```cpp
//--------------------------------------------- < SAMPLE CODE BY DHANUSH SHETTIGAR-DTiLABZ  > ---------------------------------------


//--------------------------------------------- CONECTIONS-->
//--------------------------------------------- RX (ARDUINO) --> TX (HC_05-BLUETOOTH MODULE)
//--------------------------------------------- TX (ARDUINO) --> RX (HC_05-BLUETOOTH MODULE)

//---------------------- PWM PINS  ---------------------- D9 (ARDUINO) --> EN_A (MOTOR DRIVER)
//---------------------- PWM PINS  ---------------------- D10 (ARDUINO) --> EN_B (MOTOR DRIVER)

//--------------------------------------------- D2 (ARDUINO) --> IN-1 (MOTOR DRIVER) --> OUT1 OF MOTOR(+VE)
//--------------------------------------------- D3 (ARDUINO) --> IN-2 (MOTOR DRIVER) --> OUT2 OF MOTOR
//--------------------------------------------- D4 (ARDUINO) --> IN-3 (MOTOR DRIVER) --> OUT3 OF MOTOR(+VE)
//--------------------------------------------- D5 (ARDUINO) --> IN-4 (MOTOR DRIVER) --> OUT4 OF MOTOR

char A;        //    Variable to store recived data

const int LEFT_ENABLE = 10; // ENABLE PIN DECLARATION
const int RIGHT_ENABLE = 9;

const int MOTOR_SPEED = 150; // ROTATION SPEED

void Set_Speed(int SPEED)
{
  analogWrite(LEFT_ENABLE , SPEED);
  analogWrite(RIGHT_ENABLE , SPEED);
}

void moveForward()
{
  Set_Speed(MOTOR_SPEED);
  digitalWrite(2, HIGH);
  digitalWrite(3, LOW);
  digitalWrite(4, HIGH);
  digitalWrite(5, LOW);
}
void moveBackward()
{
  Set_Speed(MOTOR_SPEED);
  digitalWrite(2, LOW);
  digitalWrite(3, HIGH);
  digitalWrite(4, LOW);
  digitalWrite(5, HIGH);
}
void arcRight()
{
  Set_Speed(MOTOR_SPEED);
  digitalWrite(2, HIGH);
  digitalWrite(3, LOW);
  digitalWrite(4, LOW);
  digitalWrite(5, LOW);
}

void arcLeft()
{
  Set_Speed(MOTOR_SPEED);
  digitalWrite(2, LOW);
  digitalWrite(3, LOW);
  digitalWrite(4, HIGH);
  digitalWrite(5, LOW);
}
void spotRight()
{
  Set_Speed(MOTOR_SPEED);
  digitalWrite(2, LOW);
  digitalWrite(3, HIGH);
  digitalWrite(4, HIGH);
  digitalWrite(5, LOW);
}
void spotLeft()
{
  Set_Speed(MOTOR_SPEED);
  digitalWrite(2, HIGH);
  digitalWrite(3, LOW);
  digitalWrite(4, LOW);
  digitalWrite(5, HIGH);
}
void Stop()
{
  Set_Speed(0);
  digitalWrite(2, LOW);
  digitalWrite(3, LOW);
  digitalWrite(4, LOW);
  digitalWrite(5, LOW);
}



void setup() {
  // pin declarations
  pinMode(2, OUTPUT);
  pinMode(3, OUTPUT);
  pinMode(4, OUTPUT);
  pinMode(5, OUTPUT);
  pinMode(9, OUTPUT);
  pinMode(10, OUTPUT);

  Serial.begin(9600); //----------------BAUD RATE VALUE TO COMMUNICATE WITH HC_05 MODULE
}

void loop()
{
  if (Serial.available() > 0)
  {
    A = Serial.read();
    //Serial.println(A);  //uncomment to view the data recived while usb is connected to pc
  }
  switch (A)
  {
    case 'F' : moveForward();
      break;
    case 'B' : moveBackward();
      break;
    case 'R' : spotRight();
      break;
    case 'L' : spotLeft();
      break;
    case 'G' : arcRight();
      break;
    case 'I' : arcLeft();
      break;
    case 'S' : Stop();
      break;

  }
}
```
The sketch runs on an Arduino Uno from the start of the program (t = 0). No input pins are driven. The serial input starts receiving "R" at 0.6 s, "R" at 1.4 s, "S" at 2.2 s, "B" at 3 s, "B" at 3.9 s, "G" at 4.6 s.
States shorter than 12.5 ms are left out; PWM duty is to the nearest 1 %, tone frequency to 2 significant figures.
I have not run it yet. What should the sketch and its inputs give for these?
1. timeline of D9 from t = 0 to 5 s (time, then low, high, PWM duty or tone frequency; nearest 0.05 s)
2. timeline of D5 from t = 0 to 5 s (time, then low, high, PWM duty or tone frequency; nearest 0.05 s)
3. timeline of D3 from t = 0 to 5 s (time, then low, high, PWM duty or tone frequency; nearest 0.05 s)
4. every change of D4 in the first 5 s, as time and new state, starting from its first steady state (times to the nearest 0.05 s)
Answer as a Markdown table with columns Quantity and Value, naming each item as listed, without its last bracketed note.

| Quantity | Value |
|---|---|
| timeline of D9 from t = 0 to 5 s | 0 s low; 0.6 s PWM 59 %; 2.2 s low; 3 s PWM 59 % |
| timeline of D5 from t = 0 to 5 s | 0 s low; 3 s high; 4.6 s low |
| timeline of D3 from t = 0 to 5 s | 0 s low; 0.6 s high; 2.2 s low; 3 s high; 4.6 s low |
| every change of D4 in the first 5 s, as time and new state, starting from its first steady state | 0 s low; 0.6 s high; 2.2 s low |
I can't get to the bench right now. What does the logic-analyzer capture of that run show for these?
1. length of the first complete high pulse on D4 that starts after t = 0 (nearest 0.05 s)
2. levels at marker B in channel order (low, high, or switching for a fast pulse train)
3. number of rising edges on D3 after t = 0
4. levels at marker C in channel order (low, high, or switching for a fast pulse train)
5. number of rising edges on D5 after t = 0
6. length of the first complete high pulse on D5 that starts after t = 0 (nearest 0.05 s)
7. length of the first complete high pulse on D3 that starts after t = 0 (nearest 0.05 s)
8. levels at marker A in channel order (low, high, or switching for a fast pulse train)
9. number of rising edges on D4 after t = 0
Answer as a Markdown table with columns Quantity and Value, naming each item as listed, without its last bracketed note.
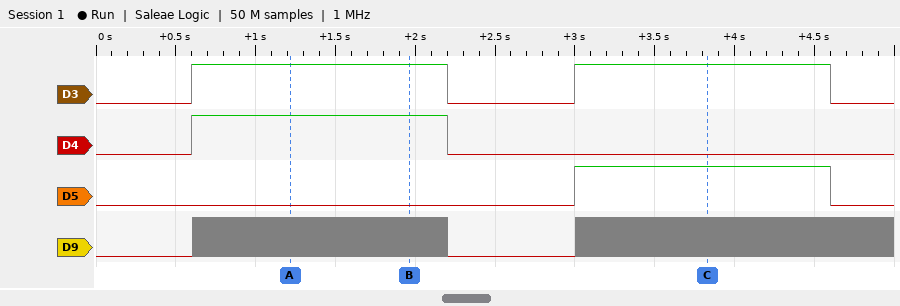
| Quantity | Value |
|---|---|
| length of the first complete high pulse on D4 that starts after t = 0 | 1.60 s |
| levels at marker B in channel order | D3 high, D4 high, D5 low, D9 switching |
| number of rising edges on D3 after t = 0 | 2 |
| levels at marker C in channel order | D3 high, D4 low, D5 high, D9 switching |
| number of rising edges on D5 after t = 0 | 1 |
| length of the first complete high pulse on D5 that starts after t = 0 | 1.60 s |
| length of the first complete high pulse on D3 that starts after t = 0 | 1.60 s |
| levels at marker A in channel order | D3 high, D4 high, D5 low, D9 switching |
| number of rising edges on D4 after t = 0 | 1 |
